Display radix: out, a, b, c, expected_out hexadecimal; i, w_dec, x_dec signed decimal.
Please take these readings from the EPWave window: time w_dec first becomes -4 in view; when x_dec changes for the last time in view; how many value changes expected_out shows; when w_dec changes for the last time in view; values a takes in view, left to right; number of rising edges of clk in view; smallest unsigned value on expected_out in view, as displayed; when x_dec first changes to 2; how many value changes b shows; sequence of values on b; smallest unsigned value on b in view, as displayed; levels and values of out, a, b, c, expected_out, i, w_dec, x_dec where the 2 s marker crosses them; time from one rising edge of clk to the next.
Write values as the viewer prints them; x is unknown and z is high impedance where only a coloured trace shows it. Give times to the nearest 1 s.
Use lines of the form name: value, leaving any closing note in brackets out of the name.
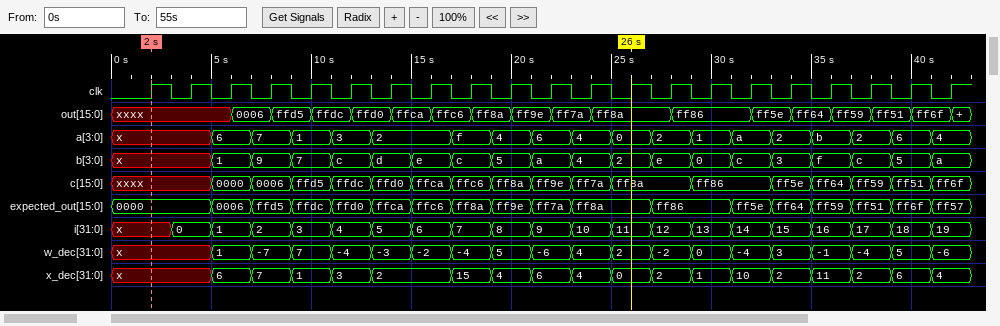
time w_dec first becomes -4 in view: 11 s
when x_dec changes for the last time in view: 41 s
how many value changes expected_out shows: 17
when w_dec changes for the last time in view: 41 s
values a takes in view, left to right: x, 6, 7, 1, 3, 2, f, 4, 6, 4, 0, 2, 1, a, 2, b, 2, 6, 4
number of rising edges of clk in view: 21
smallest unsigned value on expected_out in view, as displayed: 0000
when x_dec first changes to 2: 13 s
how many value changes b shows: 19
sequence of values on b: x, 1, 9, 7, c, d, e, c, 5, a, 4, 2, e, 0, c, 3, f, c, 5, a
smallest unsigned value on b in view, as displayed: 0
levels and values of out, a, b, c, expected_out, i, w_dec, x_dec where the 2 s marker crosses them: out=xxxx, a=x, b=x, c=xxxx, expected_out=0000, i=x, w_dec=x, x_dec=x
time from one rising edge of clk to the next: 2 s
